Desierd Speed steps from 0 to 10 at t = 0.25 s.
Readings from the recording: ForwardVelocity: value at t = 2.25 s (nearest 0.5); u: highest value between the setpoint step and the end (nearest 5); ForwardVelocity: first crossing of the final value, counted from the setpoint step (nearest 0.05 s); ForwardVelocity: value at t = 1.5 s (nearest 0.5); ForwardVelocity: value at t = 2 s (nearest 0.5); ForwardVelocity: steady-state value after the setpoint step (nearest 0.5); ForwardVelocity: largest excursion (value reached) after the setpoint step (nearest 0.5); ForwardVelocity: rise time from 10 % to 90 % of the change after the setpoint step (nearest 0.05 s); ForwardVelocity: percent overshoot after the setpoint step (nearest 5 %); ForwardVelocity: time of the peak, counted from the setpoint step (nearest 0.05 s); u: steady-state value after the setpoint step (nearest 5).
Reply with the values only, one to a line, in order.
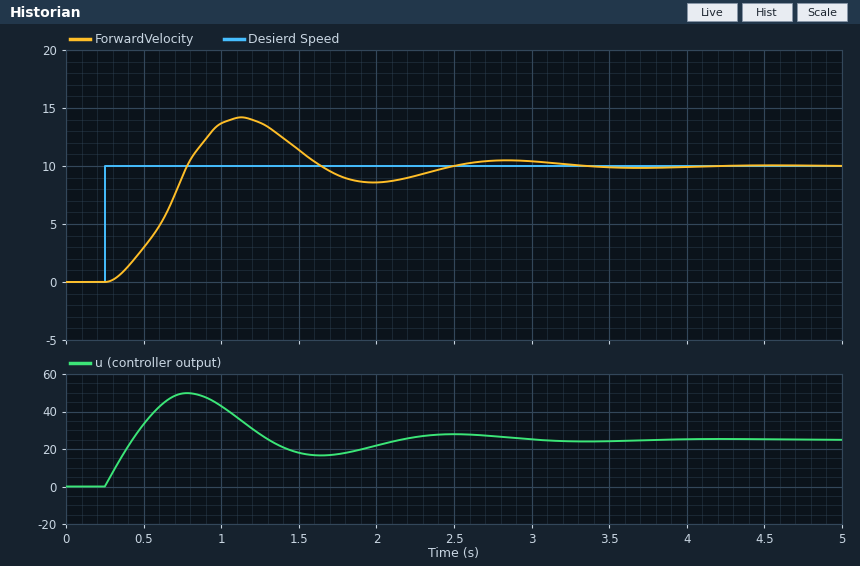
9.0
50
0.55 s
11.5
8.5
10.0
14.0
0.35 s
40 %
0.90 s
25
